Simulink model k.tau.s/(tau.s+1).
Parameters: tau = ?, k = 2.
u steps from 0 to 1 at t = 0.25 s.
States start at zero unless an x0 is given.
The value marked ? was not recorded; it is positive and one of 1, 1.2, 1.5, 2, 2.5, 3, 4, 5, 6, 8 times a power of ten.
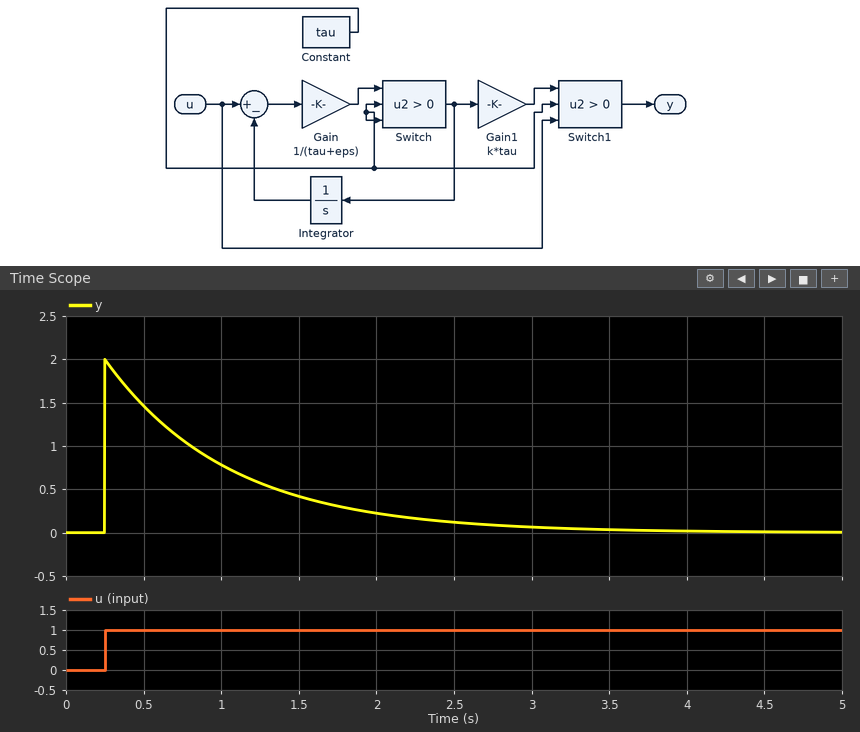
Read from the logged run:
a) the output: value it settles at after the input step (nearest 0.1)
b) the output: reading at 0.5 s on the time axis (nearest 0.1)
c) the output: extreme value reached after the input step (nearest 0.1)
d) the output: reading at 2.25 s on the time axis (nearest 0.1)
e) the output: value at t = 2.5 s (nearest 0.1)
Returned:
0.0
1.5
2.0
0.2
0.1
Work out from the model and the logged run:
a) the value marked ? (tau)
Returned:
0.8
